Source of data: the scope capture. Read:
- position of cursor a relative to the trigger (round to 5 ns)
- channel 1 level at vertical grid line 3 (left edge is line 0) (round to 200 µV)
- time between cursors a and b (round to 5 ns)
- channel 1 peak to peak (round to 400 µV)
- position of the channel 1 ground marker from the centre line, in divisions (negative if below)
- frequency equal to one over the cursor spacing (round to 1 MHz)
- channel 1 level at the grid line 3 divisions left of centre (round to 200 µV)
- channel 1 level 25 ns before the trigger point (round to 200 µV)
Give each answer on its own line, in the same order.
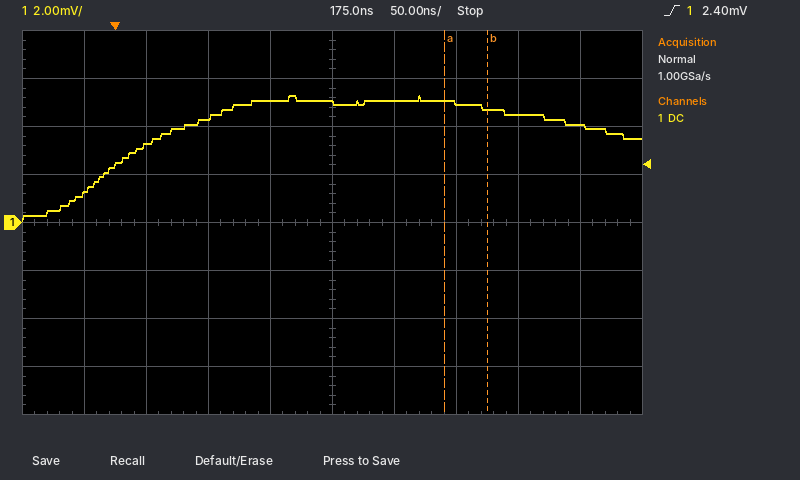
+265 ns
4.4 mV
35 ns
5.2 mV
0.0 div
29 MHz
3.2 mV
1.2 mV
